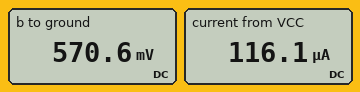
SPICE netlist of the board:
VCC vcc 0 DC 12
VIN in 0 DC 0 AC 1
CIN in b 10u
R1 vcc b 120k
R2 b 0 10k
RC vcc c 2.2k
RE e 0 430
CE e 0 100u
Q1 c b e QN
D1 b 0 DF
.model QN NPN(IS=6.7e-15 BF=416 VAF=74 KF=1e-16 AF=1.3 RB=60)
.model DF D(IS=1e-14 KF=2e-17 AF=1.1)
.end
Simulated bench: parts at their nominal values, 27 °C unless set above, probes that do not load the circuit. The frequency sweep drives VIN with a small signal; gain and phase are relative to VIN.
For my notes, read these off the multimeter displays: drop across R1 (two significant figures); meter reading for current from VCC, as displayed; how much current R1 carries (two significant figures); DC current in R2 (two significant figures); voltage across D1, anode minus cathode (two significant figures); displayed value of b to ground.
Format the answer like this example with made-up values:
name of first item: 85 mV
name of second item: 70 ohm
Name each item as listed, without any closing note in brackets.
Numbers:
drop across R1: 11 V
meter reading for current from VCC, as displayed: 116.1 µA
how much current R1 carries: 95 µA
DC current in R2: 57 µA
voltage across D1, anode minus cathode: 570 mV
displayed value of b to ground: 570.6 mV
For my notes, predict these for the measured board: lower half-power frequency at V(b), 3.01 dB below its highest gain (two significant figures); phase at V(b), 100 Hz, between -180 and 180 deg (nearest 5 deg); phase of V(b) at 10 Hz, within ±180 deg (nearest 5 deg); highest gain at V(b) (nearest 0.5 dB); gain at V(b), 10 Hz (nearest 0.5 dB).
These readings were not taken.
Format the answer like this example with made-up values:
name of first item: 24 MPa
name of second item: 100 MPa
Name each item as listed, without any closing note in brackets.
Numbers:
lower half-power frequency at V(b), 3.01 dB below its highest gain: 25 Hz
phase at V(b), 100 Hz, between -180 and 180 deg: 15 deg
phase of V(b) at 10 Hz, within ±180 deg: 70 deg
highest gain at V(b): 0 dB
gain at V(b), 10 Hz: -8.5 dB
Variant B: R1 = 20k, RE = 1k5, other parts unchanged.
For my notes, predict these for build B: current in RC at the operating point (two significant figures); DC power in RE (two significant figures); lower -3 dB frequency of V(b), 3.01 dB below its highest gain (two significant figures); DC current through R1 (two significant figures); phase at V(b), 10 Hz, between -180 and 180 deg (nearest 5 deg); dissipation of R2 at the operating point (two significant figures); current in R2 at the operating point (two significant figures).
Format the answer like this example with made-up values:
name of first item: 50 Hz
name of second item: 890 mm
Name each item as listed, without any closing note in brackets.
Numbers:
current in RC at the operating point: 39 µA
DC power in RE: 2.3 µW
lower -3 dB frequency of V(b), 3.01 dB below its highest gain: 310 Hz
DC current through R1: 570 µA
phase at V(b), 10 Hz, between -180 and 180 deg: 90 deg
dissipation of R2 at the operating point: 41 µW
current in R2 at the operating point: 64 µA
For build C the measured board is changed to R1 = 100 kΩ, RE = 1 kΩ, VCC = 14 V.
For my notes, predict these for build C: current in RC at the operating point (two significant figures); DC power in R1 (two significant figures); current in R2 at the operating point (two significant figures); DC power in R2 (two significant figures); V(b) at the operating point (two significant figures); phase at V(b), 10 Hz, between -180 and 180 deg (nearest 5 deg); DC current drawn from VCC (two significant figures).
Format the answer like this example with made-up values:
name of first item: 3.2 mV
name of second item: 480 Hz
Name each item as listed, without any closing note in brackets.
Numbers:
current in RC at the operating point: 24 µA
DC power in R1: 1.8 mW
current in R2 at the operating point: 59 µA
DC power in R2: 35 µW
V(b) at the operating point: 590 mV
phase at V(b), 10 Hz, between -180 and 180 deg: 80 deg
DC current drawn from VCC: 160 µA
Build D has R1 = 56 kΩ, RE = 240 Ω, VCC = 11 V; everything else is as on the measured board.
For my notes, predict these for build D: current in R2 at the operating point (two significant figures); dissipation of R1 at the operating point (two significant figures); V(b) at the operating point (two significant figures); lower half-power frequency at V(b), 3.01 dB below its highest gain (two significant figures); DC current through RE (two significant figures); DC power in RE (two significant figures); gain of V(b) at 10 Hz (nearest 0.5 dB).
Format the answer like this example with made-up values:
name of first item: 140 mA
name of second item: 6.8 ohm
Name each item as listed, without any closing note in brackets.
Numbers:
current in R2 at the operating point: 60 µA
dissipation of R1 at the operating point: 1.9 mW
V(b) at the operating point: 600 mV
lower half-power frequency at V(b), 3.01 dB below its highest gain: 79 Hz
DC current through RE: 57 µA
DC power in RE: 770 nW
gain of V(b) at 10 Hz: -18.0 dB
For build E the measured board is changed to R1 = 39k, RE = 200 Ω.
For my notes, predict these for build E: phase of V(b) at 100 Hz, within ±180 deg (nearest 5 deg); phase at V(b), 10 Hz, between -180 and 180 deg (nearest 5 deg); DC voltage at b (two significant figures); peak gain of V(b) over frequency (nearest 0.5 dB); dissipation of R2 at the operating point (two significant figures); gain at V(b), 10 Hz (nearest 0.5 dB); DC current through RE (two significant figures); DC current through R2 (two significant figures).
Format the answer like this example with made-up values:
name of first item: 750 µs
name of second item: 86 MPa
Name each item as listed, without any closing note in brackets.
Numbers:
phase of V(b) at 100 Hz, within ±180 deg: 55 deg
phase at V(b), 10 Hz, between -180 and 180 deg: 85 deg
DC voltage at b: 620 mV
peak gain of V(b) over frequency: 0 dB
dissipation of R2 at the operating point: 38 µW
gain at V(b), 10 Hz: -23.0 dB
DC current through RE: 89 µA
DC current through R2: 62 µA
